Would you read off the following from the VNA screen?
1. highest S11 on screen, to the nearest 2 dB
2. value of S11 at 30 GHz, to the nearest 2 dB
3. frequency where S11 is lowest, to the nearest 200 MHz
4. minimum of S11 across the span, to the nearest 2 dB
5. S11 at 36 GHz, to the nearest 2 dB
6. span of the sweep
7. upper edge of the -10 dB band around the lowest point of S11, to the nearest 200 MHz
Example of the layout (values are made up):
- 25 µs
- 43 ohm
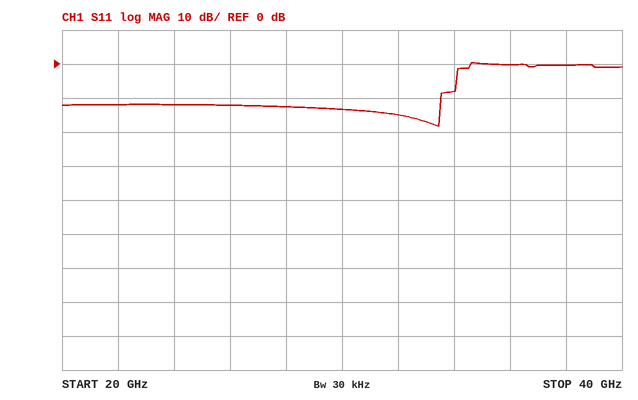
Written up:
- 0 dB
- -14 dB
- 33.4 GHz
- -18 dB
- 0 dB
- 20 GHz
- 33.6 GHz
